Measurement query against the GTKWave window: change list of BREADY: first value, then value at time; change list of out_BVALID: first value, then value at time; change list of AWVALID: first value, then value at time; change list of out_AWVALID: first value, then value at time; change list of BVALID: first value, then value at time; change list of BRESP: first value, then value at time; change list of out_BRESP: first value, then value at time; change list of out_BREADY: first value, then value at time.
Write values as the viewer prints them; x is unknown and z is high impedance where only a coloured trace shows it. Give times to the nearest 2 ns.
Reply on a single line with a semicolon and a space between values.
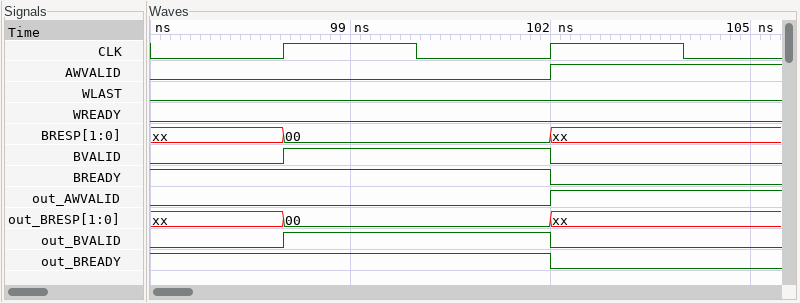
1, 0 at 102 ns; 0, 1 at 98 ns, 0 at 102 ns; 0, 1 at 102 ns; 0, 1 at 102 ns; 0, 1 at 98 ns, 0 at 102 ns; xx, 00 at 98 ns, xx at 102 ns; xx, 00 at 98 ns, xx at 102 ns; 1, 0 at 102 ns
